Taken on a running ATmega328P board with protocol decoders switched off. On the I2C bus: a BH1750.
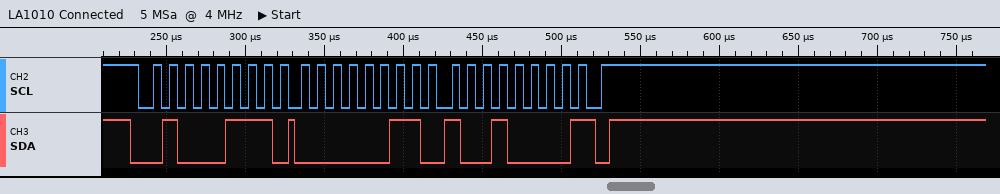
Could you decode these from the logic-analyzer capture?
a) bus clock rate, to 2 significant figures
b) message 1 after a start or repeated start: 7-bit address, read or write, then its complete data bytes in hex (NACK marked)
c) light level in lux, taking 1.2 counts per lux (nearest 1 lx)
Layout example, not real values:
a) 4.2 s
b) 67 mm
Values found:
a) 100 kHz
b) 0x23 read: 03 90 NACK
c) 760 lx
